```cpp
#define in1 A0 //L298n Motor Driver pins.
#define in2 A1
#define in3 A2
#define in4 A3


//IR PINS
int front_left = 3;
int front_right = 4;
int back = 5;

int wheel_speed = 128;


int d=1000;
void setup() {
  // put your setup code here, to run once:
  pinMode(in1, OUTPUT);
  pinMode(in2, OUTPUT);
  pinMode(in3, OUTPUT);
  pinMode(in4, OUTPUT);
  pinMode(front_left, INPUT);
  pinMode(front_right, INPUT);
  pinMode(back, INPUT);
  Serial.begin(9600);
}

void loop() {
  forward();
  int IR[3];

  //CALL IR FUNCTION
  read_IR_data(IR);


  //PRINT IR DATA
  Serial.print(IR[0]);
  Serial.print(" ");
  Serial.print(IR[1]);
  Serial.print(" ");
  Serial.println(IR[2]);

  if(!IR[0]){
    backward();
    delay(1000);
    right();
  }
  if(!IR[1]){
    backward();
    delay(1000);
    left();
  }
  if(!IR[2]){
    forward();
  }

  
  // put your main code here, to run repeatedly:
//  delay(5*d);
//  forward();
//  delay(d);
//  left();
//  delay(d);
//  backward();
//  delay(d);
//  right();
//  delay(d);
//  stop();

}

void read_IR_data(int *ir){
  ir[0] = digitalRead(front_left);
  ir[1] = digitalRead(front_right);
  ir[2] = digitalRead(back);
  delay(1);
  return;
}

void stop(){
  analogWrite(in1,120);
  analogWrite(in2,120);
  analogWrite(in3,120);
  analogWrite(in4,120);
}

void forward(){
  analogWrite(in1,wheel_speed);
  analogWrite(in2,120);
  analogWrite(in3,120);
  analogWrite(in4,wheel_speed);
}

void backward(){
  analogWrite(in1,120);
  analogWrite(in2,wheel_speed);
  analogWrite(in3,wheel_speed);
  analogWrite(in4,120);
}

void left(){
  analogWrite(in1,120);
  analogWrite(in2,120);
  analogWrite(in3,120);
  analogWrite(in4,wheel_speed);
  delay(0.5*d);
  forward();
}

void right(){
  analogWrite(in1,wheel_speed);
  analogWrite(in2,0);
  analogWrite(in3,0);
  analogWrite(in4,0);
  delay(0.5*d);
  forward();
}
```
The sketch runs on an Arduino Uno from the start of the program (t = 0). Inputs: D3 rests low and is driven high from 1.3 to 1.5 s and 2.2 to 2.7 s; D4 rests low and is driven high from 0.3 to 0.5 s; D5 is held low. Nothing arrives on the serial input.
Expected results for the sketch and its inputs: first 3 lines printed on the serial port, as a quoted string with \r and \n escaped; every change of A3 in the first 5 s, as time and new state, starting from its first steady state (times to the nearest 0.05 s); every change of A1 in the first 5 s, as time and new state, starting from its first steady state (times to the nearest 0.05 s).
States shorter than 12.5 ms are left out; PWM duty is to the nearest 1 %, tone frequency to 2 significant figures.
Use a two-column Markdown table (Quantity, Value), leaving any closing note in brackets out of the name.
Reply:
| Quantity | Value |
|---|---|
| first 3 lines printed on the serial port, as a quoted string with \r and \n escaped | "0 0 0\r\n0 0 0\r\n0 0 0\r\n" |
| every change of A3 in the first 5 s, as time and new state, starting from its first steady state | 0 s low; 2.5 s high; 3 s low |
| every change of A1 in the first 5 s, as time and new state, starting from its first steady state | 0 s high; 1 s low; 1.5 s high; 2.5 s low; 3 s high; 4 s low; 4.5 s high |
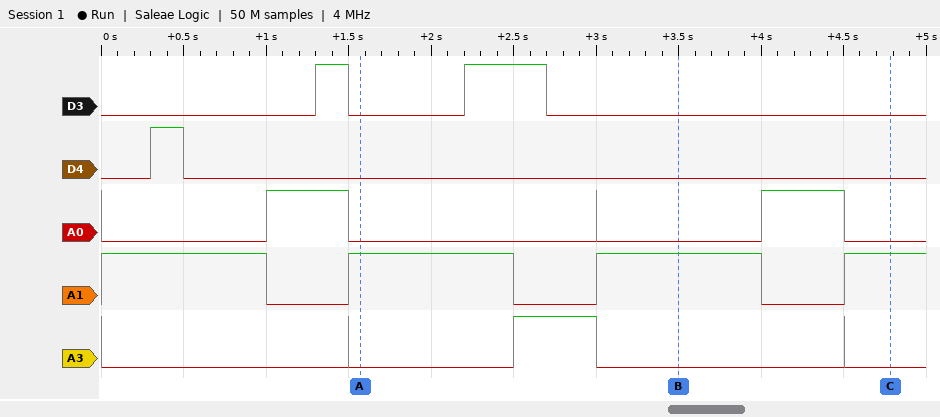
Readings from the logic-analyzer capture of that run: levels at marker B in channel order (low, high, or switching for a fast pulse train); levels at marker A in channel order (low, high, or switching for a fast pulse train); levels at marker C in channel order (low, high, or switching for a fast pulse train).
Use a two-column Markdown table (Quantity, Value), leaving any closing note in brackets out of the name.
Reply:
| Quantity | Value |
|---|---|
| levels at marker B in channel order | D3 low, D4 low, A0 low, A1 high, A3 low |
| levels at marker A in channel order | D3 low, D4 low, A0 low, A1 high, A3 low |
| levels at marker C in channel order | D3 low, D4 low, A0 low, A1 high, A3 low |
